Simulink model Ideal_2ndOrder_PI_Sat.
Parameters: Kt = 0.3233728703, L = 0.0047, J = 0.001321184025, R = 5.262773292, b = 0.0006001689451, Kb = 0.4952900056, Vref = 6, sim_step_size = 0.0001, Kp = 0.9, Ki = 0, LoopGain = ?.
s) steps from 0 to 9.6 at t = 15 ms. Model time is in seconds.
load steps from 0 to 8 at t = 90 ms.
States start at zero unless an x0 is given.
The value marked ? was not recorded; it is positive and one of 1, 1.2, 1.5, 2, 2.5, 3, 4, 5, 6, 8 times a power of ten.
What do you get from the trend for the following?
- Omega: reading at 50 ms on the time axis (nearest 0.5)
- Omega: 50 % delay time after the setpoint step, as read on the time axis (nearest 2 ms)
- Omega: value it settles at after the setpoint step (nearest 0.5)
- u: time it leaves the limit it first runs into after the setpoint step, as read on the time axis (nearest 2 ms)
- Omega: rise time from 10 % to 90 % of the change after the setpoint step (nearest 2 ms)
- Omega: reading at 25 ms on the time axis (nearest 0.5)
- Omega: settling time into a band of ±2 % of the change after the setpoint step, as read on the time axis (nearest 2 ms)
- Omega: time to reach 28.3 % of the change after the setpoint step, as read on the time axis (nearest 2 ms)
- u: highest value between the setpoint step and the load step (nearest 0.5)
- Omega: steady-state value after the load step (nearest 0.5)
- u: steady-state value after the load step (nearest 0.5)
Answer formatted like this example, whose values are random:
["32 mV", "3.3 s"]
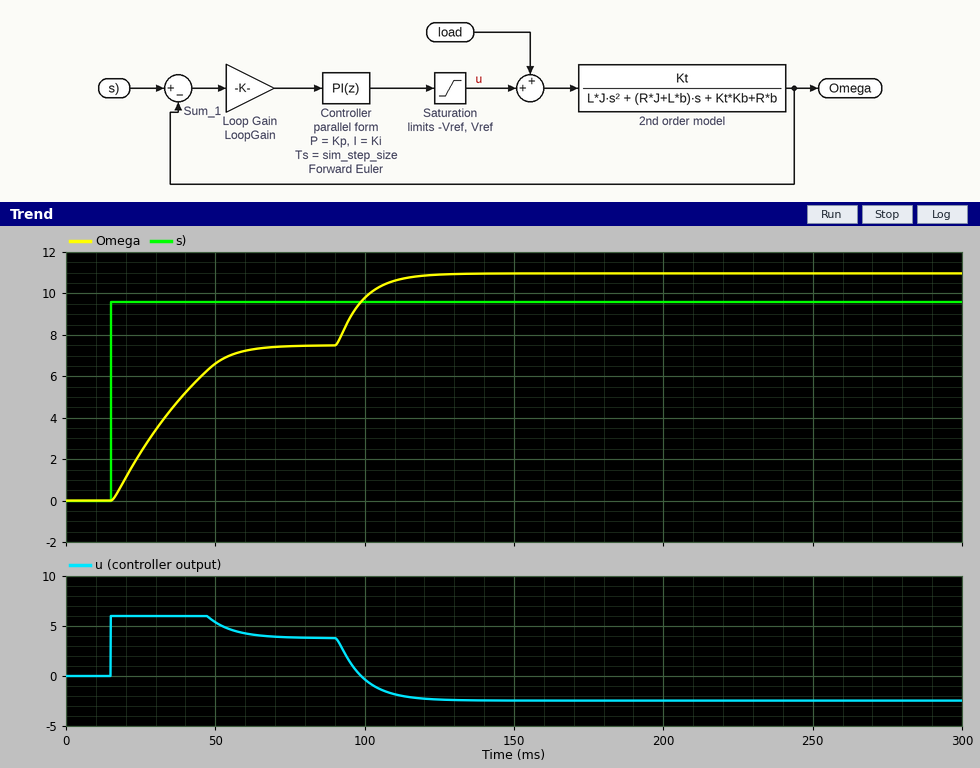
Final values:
["6.5", "32 ms", "7.5", "48 ms", "32 ms", "2.5", "64 ms", "24 ms", "6.0", "11.0", "-2.5"]
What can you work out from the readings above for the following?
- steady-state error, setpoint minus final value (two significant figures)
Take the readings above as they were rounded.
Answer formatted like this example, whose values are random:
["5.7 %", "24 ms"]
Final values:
["2.1"]
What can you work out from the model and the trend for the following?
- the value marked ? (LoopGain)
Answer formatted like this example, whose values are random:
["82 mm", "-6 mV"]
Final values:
["2"]
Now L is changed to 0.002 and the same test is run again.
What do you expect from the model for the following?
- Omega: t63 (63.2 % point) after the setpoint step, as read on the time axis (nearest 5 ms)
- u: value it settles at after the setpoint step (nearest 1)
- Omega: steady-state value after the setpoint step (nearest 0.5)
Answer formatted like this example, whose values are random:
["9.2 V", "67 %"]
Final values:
["35 ms", "4", "7.5"]
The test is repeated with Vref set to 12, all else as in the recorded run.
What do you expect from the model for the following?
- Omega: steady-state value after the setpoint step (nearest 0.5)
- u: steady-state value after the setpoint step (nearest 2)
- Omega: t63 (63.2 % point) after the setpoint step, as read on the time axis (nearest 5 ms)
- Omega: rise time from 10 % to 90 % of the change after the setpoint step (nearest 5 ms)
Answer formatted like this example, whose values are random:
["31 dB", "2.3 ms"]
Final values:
["7.5", "4", "25 ms", "20 ms"]
